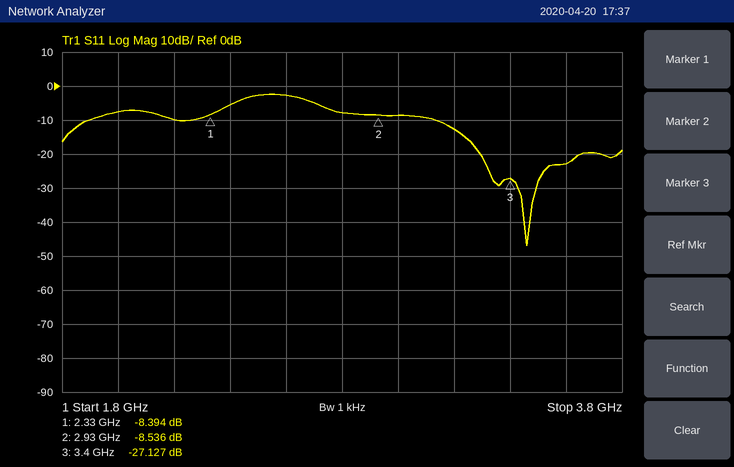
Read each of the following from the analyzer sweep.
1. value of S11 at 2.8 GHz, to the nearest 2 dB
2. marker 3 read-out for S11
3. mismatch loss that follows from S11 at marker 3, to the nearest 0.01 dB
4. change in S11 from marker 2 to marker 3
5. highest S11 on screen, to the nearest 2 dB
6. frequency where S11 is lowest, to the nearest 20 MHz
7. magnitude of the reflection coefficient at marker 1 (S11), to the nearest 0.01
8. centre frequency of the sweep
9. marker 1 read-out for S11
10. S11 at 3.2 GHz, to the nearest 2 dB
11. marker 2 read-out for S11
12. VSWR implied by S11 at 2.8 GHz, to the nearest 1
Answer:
-8 dB
-27.127 dB
0.01 dB
-18.591 dB
-2 dB
3.46 GHz
0.38
2.8 GHz
-8.394 dB
-12 dB
-8.536 dB
2
